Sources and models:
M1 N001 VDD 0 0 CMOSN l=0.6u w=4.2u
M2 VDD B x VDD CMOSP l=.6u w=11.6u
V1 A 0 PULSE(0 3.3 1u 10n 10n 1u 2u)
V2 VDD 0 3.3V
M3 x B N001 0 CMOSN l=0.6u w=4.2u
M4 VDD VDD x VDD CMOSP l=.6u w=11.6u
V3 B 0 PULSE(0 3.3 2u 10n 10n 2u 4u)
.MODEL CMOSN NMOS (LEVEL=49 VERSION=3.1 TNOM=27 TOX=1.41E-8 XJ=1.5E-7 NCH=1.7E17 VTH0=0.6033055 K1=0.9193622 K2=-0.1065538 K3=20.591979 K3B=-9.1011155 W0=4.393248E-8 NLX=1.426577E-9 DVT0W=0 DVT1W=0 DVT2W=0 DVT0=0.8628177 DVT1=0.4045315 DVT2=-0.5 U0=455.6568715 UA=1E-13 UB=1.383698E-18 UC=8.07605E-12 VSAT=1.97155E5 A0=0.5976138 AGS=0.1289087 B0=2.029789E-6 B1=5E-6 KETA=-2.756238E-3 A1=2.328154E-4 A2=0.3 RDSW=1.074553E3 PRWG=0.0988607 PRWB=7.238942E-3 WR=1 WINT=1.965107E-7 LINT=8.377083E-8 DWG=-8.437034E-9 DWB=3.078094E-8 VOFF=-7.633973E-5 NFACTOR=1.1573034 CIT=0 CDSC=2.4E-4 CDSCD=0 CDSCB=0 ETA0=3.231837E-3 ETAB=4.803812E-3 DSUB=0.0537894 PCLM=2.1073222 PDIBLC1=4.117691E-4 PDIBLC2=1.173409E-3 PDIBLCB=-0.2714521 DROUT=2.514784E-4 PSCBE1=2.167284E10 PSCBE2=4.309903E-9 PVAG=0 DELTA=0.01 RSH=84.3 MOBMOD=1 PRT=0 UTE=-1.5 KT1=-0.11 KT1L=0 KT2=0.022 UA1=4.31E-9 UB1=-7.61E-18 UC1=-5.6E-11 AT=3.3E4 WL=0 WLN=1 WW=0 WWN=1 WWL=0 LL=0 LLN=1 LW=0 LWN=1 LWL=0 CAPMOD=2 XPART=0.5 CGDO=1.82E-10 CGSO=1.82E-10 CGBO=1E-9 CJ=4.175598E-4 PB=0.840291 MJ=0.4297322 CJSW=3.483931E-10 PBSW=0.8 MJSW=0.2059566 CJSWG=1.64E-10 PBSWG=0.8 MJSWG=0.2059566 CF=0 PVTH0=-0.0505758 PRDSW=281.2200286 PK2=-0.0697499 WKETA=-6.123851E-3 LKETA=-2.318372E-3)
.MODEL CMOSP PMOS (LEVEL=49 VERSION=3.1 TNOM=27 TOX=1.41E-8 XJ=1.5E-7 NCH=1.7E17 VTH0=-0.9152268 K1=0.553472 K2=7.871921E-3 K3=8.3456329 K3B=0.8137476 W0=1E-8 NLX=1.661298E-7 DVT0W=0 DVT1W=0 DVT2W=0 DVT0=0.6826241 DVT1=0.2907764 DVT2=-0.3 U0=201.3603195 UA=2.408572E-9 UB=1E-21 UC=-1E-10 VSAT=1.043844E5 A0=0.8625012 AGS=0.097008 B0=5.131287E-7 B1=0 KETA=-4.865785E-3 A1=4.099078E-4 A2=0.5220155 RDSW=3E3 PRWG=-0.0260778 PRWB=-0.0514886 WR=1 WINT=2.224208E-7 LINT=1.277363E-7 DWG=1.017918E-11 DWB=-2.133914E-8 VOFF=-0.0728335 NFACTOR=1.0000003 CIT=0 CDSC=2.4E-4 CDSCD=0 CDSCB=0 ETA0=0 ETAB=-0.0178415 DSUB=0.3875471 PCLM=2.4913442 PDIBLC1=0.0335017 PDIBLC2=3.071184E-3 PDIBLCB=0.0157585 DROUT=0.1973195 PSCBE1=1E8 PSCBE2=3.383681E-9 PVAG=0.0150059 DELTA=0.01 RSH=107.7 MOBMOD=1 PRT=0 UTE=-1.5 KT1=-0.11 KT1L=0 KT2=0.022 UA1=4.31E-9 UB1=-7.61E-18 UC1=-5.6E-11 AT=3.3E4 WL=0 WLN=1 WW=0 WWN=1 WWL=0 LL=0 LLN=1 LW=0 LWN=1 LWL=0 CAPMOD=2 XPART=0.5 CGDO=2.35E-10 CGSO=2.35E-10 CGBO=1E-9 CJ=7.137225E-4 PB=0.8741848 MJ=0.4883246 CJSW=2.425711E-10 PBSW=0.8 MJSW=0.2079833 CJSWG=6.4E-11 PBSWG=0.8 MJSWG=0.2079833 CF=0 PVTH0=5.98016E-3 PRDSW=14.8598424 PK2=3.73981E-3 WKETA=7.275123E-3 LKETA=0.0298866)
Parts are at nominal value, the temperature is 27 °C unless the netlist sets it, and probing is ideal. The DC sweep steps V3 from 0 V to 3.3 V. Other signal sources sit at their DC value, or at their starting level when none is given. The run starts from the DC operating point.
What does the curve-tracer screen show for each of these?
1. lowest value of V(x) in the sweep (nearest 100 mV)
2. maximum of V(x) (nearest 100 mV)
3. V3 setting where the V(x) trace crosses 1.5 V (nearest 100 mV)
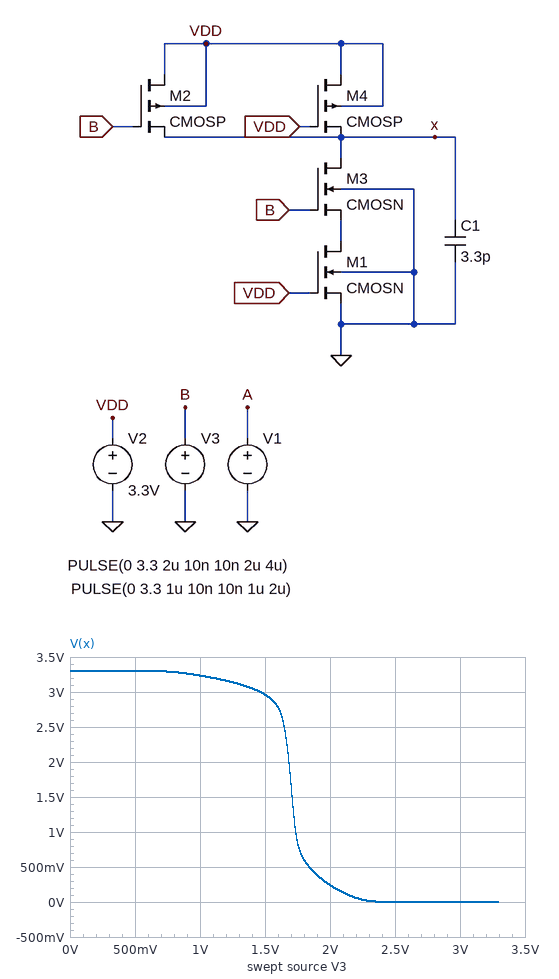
0 V
3.3 V
1.7 V
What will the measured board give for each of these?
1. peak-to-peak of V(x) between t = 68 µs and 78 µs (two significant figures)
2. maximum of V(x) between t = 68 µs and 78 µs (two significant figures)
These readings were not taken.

3.3 V
3.3 V
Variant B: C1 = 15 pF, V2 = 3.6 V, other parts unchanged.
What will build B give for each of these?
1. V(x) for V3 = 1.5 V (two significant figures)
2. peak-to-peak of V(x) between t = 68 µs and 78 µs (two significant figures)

3.3 V
3.6 V
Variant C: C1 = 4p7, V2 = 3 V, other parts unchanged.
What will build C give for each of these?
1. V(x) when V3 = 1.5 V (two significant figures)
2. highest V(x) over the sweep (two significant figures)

1.6 V
3.0 V
